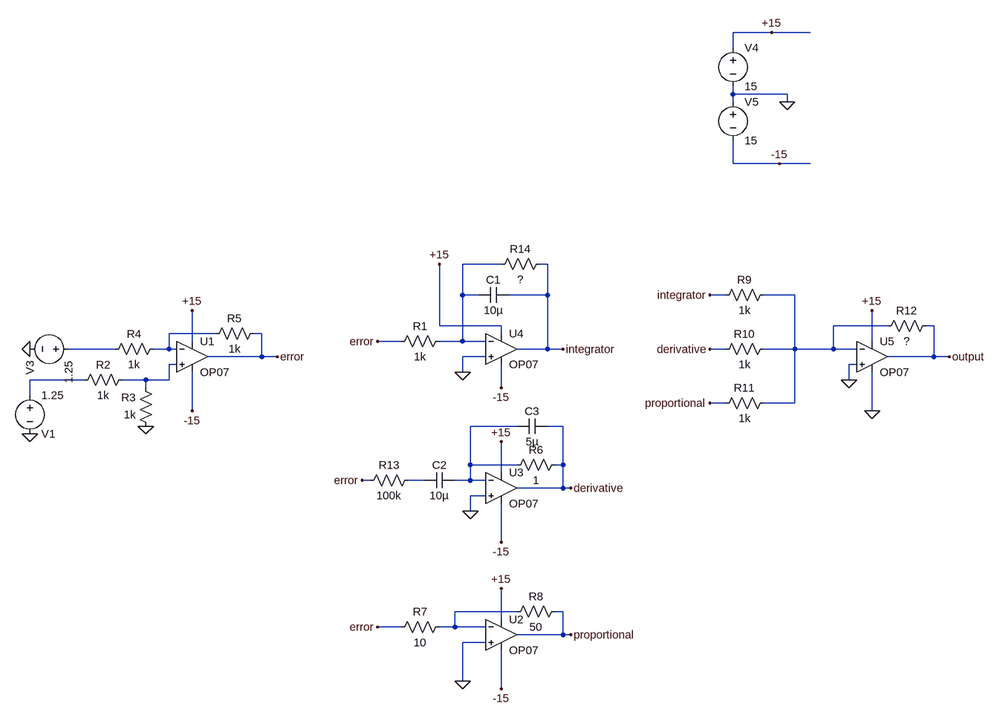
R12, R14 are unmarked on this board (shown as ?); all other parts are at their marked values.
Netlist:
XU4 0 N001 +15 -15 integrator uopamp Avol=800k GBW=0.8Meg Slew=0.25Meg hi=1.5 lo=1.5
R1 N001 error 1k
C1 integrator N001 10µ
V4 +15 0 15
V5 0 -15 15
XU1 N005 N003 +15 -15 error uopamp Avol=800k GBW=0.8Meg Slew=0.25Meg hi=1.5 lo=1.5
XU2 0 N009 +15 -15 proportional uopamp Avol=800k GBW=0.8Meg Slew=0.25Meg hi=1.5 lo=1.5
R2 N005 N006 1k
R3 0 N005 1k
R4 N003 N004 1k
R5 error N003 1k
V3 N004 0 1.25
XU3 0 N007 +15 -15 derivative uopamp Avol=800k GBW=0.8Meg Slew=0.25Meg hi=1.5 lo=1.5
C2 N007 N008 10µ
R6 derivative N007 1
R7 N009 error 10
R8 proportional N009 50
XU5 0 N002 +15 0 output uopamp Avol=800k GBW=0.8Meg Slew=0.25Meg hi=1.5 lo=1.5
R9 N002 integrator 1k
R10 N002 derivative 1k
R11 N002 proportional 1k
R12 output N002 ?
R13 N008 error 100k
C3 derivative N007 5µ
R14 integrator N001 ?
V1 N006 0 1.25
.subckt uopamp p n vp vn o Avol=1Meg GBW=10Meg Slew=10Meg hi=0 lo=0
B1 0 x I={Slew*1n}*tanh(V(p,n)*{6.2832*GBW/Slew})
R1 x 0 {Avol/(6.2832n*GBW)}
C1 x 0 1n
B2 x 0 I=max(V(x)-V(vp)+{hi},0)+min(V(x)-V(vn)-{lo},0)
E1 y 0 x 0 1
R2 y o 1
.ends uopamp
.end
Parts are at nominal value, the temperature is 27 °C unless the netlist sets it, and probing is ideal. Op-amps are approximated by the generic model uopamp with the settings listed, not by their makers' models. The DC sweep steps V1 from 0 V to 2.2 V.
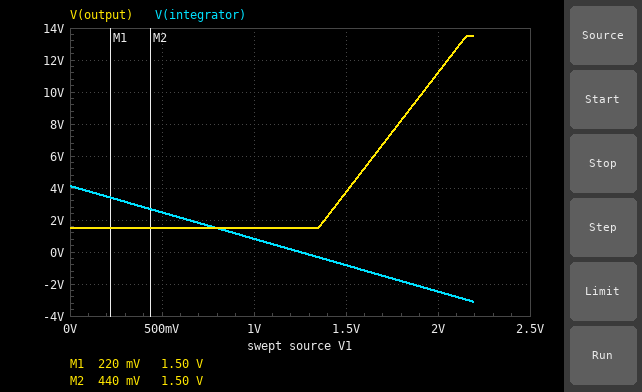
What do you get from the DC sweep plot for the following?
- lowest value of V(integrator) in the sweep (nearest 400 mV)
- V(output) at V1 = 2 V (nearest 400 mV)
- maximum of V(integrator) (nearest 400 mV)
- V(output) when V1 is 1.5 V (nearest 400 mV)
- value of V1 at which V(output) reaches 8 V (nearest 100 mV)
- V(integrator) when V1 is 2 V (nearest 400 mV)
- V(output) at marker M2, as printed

-3.2 V
11.2 V
4.0 V
3.6 V
1.8 V
-2.4 V
1.50 V
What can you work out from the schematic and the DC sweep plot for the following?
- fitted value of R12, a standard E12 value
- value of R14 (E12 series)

1.8 kΩ
3.3 kΩ
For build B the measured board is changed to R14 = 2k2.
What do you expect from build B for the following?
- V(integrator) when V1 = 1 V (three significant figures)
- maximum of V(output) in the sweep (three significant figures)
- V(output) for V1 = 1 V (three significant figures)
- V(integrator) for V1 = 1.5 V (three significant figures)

550 mV
12.3 V
1.50 V
-550 mV
